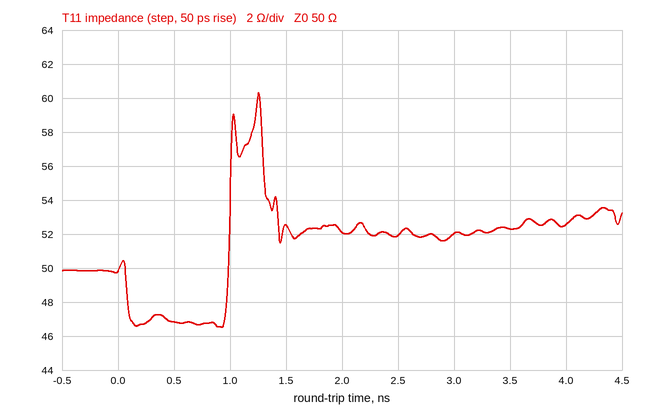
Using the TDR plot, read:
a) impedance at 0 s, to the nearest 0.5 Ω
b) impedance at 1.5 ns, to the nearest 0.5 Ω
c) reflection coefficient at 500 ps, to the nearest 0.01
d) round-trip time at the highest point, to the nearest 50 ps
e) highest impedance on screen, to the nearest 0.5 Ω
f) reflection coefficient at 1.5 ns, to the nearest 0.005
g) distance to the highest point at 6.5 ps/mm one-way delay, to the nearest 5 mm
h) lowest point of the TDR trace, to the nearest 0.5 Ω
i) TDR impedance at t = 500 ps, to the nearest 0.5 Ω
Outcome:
50.0 Ω
52.5 Ω
-0.03
1.25 ns
60.5 Ω
+0.025
95 mm
46.5 Ω
47.0 Ω
